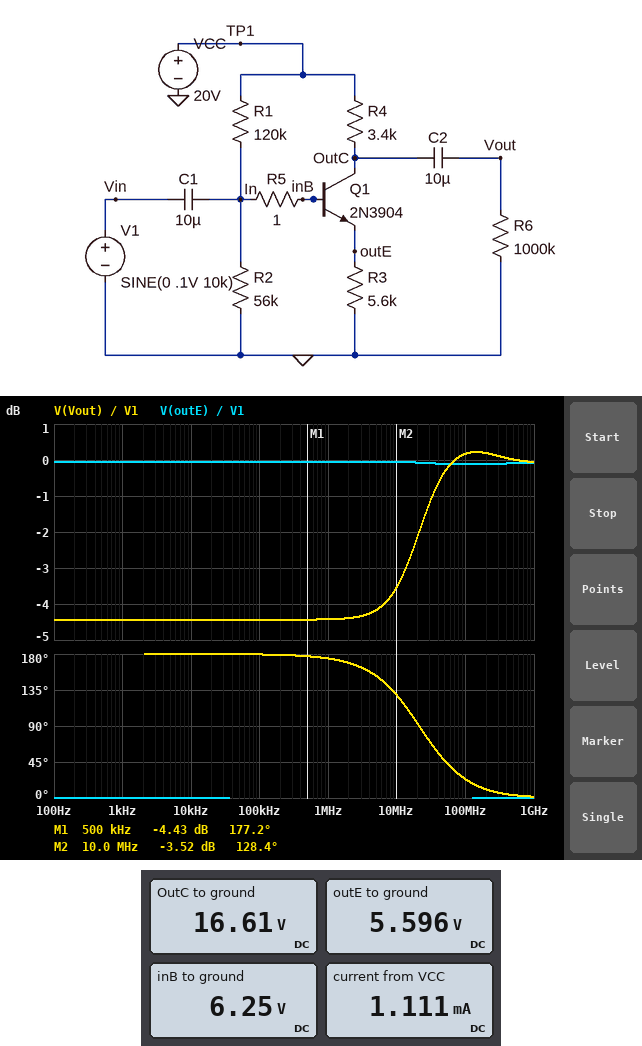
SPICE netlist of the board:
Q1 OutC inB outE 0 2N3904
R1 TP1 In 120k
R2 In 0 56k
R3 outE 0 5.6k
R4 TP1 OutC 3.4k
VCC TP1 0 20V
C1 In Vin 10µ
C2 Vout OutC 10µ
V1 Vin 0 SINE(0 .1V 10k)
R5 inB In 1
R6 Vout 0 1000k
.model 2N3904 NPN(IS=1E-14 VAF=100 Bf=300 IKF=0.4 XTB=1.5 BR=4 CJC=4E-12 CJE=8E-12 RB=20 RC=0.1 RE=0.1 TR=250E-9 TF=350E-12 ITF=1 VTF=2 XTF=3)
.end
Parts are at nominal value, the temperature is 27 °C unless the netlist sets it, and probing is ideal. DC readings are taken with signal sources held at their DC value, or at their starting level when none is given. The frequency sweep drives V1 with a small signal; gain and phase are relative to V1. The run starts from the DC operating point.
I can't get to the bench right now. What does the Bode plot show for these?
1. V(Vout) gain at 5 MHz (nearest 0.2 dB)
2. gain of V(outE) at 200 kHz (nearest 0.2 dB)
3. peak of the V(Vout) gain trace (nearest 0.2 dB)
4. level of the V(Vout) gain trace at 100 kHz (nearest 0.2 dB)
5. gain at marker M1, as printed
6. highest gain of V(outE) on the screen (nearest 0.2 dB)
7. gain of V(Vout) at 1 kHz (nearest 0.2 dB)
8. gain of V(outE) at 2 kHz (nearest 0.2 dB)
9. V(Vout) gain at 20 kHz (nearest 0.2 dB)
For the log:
-4.2 dB
0 dB
0.2 dB
-4.4 dB
-4.43 dB
0 dB
-4.4 dB
0 dB
-4.4 dB
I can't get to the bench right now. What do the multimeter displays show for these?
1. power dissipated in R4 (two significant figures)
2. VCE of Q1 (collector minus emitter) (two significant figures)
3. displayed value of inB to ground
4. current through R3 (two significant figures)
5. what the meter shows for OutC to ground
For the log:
3.4 mW
11 V
6.25 V
1.0 mA
16.61 V
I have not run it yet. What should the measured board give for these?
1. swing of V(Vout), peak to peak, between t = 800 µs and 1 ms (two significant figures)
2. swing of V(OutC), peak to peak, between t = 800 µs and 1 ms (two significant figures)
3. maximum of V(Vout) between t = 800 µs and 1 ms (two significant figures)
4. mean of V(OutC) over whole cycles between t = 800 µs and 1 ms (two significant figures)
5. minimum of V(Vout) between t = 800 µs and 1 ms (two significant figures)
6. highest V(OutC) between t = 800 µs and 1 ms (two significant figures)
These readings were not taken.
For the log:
120 mV
120 mV
60 mV
17 V
-60 mV
17 V
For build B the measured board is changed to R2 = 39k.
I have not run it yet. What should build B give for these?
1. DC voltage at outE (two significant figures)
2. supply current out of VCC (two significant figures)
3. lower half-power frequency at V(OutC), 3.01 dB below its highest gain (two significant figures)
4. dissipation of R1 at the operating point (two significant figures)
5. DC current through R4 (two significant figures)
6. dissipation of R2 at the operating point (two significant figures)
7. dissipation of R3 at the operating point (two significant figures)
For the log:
4.2 V
870 µA
16 MHz
1.9 mW
750 µA
600 µW
3.1 mW
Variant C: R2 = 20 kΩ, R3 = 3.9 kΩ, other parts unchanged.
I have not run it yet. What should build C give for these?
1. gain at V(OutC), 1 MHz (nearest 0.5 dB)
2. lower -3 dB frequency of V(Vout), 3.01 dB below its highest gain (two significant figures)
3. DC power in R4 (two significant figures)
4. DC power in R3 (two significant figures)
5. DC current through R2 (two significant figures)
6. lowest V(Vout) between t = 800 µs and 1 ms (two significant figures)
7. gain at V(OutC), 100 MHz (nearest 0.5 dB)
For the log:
-1.5 dB
1.8 Hz
1.1 mW
1.2 mW
140 µA
-86 mV
0.5 dB
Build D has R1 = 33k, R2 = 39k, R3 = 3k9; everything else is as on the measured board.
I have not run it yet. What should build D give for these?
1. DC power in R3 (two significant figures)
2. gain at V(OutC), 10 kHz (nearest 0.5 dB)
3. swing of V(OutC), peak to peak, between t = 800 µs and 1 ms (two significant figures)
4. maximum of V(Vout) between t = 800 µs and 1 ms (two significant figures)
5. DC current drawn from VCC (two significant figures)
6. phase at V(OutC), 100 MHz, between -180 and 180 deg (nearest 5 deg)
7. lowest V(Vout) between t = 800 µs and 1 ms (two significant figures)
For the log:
26 mW
-1.5 dB
170 mV
86 mV
2.8 mA
15 deg
-86 mV
